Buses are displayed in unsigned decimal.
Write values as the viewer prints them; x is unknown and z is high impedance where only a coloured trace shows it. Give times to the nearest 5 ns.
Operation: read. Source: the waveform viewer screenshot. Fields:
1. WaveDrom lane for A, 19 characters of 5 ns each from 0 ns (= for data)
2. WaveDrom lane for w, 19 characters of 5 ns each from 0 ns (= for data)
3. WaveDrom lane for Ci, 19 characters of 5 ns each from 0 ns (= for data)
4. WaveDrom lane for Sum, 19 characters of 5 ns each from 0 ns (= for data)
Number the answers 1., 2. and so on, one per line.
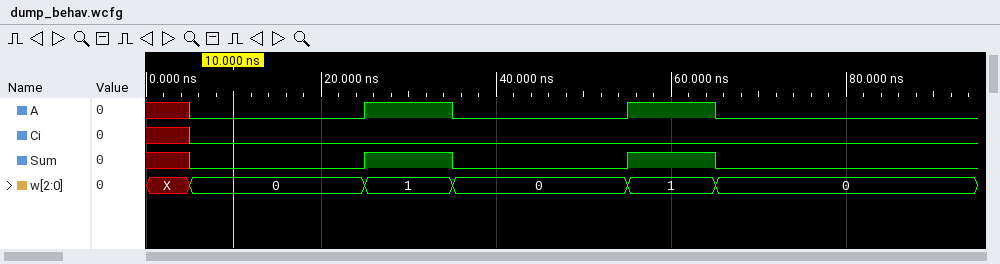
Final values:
1. {name: 'A', wave: 'x0...1.0...1.0.....'}
2. {name: 'w', wave: '==...=.=...=.=.....', data: 'X 0 1 0 1 0'}
3. {name: 'Ci', wave: 'x0.................'}
4. {name: 'Sum', wave: 'x0...1.0...1.0.....'}
